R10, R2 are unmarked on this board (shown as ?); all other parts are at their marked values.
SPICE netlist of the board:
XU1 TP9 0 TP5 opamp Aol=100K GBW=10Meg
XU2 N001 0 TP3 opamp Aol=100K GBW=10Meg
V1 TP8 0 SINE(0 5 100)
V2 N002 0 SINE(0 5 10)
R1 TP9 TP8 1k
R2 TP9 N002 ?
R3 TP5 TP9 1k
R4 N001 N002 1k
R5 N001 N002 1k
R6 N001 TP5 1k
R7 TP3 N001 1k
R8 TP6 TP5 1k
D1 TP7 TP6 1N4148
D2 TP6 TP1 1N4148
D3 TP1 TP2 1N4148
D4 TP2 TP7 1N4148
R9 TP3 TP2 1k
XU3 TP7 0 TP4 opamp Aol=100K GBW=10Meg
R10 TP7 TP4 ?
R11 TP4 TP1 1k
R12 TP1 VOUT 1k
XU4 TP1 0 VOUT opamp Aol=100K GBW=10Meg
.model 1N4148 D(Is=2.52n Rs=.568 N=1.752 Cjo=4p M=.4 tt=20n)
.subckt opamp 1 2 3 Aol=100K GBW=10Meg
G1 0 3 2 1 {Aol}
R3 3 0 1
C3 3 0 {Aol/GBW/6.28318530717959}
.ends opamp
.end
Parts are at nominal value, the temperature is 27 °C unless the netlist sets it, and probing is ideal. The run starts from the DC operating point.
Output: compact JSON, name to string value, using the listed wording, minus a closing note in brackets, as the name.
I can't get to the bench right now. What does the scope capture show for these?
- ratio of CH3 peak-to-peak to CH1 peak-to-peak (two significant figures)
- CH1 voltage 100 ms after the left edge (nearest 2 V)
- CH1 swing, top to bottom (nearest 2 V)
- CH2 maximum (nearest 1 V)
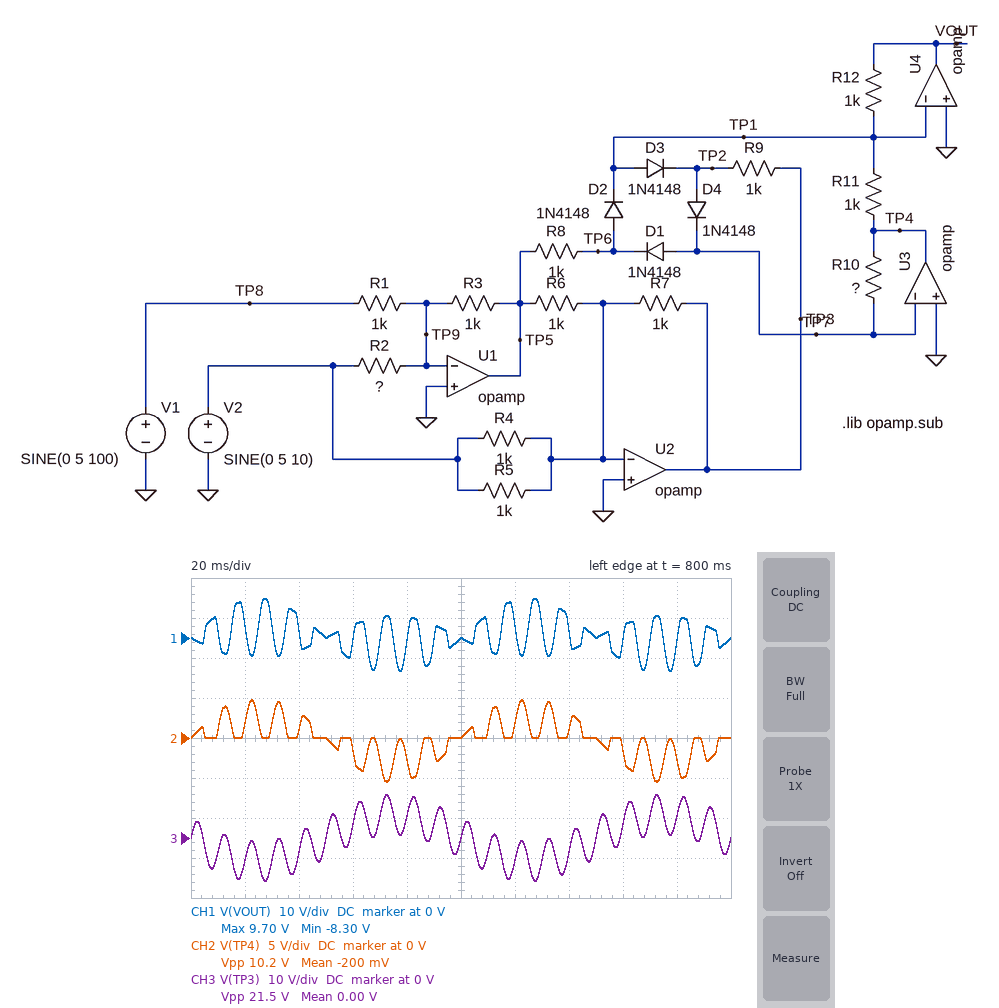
{"ratio of CH3 peak-to-peak to CH1 peak-to-peak": "1.2", "CH1 voltage 100 ms after the left edge": "0 V", "CH1 swing, top to bottom": "18 V", "CH2 maximum": "5 V"}
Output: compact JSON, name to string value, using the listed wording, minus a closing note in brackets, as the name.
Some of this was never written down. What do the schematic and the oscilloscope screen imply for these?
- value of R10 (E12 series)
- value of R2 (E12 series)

{"value of R10": "560 Ω", "value of R2": "1.2 kΩ"}
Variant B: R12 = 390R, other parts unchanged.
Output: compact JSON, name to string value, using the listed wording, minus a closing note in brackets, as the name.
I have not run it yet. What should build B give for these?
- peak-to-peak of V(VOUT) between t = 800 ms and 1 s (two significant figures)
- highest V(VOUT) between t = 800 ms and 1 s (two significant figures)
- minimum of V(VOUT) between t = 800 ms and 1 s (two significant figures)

{"peak-to-peak of V(VOUT) between t = 800 ms and 1 s": "7.0 V", "highest V(VOUT) between t = 800 ms and 1 s": "3.8 V", "minimum of V(VOUT) between t = 800 ms and 1 s": "-3.2 V"}
